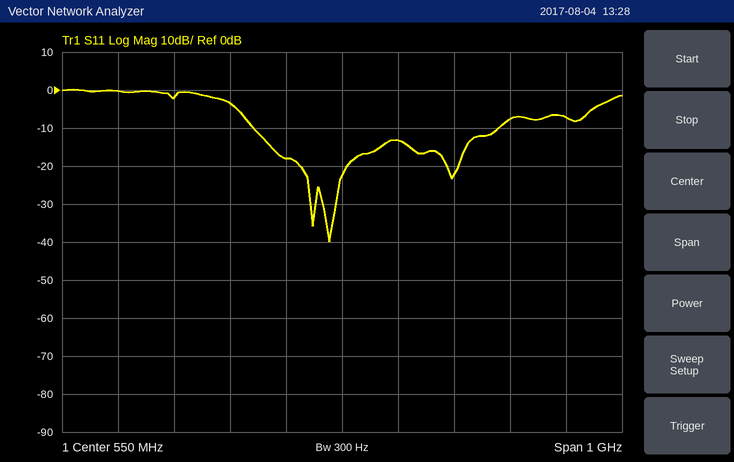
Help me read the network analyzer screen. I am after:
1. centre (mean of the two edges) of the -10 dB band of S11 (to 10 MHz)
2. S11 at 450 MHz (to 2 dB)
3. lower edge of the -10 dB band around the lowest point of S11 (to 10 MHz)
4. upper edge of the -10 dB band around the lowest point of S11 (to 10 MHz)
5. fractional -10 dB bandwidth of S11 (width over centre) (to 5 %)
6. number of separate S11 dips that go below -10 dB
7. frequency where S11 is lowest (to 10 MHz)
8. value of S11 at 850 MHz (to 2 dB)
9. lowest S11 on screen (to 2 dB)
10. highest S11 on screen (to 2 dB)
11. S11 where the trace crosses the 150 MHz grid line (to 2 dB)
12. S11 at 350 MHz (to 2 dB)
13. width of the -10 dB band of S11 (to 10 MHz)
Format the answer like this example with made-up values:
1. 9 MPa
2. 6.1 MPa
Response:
1. 610 MHz
2. -18 dB
3. 390 MHz
4. 830 MHz
5. 70 %
6. 3
7. 530 MHz
8. -8 dB
9. -40 dB
10. 0 dB
11. 0 dB
12. -4 dB
13. 440 MHz
